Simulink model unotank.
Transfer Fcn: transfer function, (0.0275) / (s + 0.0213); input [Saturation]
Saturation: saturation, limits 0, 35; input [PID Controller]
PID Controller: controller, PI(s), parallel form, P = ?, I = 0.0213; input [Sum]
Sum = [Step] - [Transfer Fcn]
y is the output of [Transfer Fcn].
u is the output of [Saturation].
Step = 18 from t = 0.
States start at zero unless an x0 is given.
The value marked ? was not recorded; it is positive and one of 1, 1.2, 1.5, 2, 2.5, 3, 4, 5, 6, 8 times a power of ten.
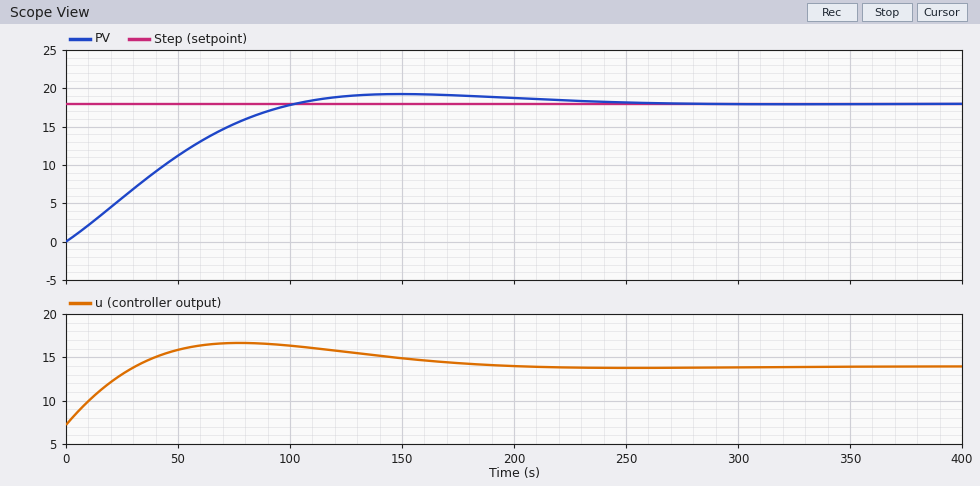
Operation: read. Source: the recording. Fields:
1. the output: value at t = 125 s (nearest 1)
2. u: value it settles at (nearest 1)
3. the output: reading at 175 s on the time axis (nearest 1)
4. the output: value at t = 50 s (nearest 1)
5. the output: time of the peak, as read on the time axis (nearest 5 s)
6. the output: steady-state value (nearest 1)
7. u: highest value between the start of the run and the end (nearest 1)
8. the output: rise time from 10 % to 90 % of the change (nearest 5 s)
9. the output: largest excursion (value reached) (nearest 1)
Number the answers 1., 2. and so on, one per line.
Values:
1. 19
2. 14
3. 19
4. 11
5. 150 s
6. 18
7. 17
8. 75 s
9. 19
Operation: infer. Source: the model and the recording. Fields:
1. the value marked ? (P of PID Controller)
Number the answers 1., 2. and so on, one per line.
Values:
1. 0.4
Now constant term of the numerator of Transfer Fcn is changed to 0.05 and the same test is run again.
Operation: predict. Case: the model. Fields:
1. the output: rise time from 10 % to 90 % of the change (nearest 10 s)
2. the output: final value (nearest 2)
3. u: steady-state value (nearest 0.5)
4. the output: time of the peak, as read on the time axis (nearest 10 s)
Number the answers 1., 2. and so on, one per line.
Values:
1. 50 s
2. 18
3. 7.5
4. 100 s
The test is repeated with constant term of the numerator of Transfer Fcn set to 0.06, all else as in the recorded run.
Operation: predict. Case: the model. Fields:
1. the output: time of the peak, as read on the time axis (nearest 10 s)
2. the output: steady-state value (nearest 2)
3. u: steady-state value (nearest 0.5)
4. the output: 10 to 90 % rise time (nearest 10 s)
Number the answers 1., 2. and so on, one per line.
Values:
1. 90 s
2. 18
3. 6.5
4. 40 s
